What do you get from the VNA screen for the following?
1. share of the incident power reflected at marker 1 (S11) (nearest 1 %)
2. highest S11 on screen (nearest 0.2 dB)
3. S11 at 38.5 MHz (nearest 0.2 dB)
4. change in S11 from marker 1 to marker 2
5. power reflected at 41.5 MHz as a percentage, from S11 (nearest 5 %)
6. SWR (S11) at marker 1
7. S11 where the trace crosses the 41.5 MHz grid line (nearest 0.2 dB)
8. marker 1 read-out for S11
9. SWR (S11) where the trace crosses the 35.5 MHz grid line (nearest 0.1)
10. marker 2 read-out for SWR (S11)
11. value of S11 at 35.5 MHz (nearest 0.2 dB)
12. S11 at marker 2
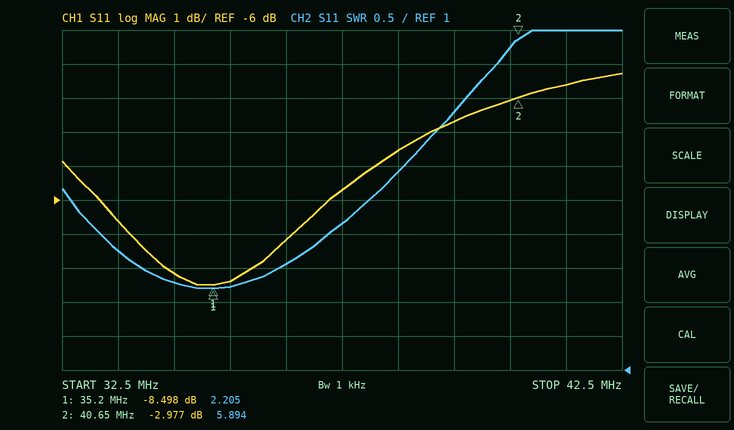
14 %
-2.2 dB
-4.6 dB
5.521 dB
55 %
2.205
-2.6 dB
-8.498 dB
2.2
5.894
-8.4 dB
-2.977 dB
